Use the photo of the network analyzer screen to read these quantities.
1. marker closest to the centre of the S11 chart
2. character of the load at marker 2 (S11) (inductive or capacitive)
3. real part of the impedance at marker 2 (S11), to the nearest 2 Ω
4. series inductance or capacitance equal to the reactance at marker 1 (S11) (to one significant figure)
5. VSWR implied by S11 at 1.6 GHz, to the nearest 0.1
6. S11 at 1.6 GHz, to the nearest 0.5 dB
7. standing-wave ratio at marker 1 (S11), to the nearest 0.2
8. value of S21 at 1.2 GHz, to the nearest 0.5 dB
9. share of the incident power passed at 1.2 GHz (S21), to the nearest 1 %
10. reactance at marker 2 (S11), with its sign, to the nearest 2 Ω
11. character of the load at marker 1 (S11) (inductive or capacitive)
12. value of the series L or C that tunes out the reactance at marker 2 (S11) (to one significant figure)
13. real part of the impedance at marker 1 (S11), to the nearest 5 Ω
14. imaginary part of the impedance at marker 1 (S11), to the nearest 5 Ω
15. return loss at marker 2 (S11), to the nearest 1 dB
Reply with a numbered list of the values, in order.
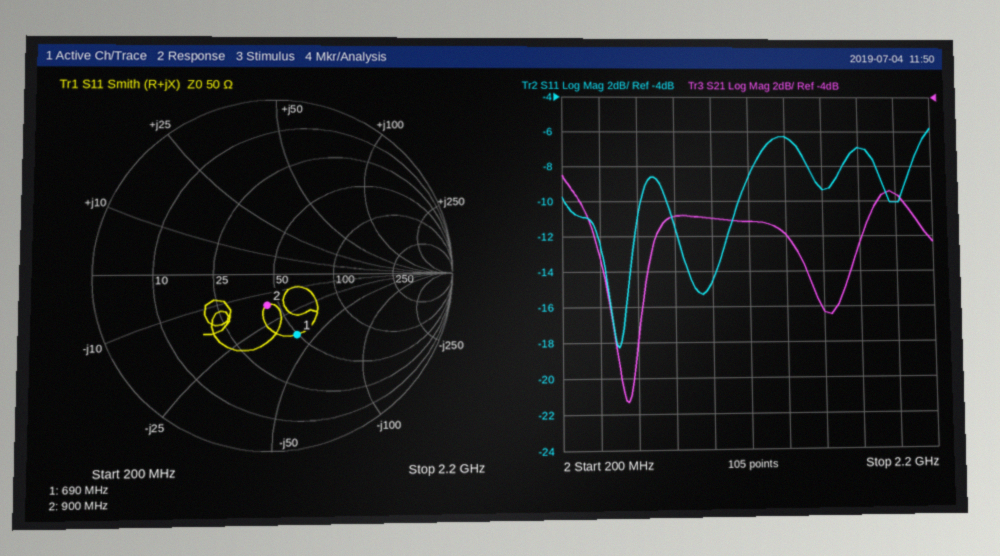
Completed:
1. marker 2
2. capacitive
3. 44 Ω
4. 6 pF
5. 2.0
6. -9.5 dB
7. 2.2
8. -11.0 dB
9. 8 %
10. -16 Ω
11. capacitive
12. 3 nH
13. 50 Ω
14. -40 Ω
15. 15 dB
